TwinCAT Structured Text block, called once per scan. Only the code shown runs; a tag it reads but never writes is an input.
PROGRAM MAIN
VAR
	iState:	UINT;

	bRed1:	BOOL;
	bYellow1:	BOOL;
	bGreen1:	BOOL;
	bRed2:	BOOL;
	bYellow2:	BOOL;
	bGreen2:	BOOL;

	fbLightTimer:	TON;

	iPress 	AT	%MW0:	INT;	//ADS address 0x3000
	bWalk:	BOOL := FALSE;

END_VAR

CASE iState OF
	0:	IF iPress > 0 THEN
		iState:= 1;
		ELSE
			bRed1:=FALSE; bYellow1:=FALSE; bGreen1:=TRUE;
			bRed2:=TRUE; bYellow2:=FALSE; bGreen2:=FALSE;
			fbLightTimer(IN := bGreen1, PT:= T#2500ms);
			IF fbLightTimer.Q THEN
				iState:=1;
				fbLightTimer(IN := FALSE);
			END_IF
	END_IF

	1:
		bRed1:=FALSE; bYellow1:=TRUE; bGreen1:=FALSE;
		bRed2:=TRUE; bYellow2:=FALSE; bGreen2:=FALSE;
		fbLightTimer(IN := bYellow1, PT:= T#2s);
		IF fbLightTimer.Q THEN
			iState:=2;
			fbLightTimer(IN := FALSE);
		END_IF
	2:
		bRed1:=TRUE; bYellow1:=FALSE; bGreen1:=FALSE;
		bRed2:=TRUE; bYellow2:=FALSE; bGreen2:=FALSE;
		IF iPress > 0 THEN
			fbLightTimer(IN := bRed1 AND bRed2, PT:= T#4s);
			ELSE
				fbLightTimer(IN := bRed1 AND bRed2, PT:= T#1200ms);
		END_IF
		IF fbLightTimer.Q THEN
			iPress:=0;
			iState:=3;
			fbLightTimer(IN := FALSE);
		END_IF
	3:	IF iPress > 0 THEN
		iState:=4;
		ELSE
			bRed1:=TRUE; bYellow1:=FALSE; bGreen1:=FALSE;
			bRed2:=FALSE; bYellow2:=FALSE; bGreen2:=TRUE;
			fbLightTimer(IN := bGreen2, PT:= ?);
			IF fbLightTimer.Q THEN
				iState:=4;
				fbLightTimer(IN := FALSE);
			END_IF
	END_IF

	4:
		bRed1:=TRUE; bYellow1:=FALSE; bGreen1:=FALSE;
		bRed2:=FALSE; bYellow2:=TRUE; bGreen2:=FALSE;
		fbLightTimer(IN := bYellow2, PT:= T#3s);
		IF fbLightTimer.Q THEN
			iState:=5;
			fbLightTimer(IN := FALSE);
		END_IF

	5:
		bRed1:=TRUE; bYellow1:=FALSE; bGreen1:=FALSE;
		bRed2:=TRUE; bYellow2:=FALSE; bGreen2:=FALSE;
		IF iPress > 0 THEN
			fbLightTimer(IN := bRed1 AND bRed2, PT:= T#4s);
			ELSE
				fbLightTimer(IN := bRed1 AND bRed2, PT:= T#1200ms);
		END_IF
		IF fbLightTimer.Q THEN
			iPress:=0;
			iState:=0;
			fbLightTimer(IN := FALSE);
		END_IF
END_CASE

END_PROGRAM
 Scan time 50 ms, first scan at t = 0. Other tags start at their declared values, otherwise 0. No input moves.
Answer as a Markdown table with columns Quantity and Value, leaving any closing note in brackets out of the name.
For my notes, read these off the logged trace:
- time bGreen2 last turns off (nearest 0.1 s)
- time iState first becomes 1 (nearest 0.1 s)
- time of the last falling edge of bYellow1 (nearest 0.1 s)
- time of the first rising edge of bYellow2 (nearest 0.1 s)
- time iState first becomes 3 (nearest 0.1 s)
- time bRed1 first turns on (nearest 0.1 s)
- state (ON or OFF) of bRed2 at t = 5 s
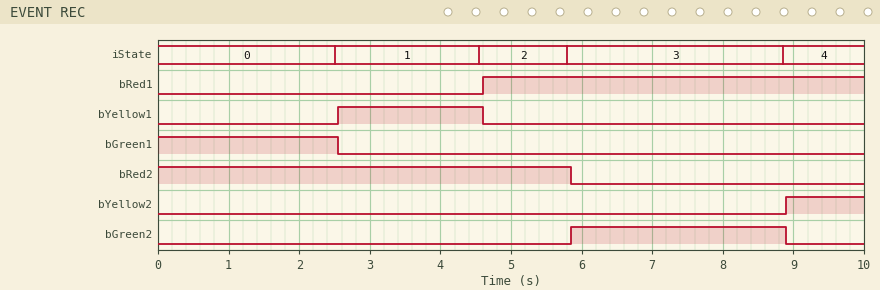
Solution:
| Quantity | Value |
|---|---|
| time bGreen2 last turns off | 8.9 s |
| time iState first becomes 1 | 2.5 s |
| time of the last falling edge of bYellow1 | 4.6 s |
| time of the first rising edge of bYellow2 | 8.9 s |
| time iState first becomes 3 | 5.8 s |
| time bRed1 first turns on | 4.6 s |
| state (ON or OFF) of bRed2 at t = 5 s | ON |
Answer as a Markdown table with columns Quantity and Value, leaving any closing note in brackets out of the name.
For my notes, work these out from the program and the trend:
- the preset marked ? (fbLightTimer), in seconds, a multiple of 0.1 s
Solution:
| Quantity | Value |
|---|---|
| the preset marked ? (fbLightTimer), in seconds, a multiple of 0.1 s | 3.0 s |
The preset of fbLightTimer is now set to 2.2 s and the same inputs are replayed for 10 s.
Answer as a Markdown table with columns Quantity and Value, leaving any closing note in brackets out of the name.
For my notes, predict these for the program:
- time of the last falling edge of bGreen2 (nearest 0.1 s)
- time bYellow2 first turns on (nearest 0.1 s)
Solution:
| Quantity | Value |
|---|---|
| time of the last falling edge of bGreen2 | 8.1 s |
| time bYellow2 first turns on | 8.1 s |
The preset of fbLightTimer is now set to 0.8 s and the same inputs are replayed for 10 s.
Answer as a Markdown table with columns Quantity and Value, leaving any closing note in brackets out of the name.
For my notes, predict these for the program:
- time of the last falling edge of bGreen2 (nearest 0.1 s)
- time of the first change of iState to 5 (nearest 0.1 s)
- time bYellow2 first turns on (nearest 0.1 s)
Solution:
| Quantity | Value |
|---|---|
| time of the last falling edge of bGreen2 | 6.7 s |
| time of the first change of iState to 5 | 9.7 s |
| time bYellow2 first turns on | 6.7 s |
